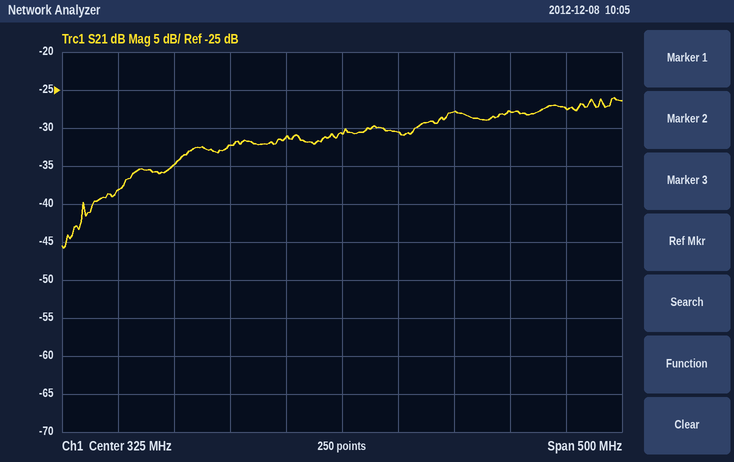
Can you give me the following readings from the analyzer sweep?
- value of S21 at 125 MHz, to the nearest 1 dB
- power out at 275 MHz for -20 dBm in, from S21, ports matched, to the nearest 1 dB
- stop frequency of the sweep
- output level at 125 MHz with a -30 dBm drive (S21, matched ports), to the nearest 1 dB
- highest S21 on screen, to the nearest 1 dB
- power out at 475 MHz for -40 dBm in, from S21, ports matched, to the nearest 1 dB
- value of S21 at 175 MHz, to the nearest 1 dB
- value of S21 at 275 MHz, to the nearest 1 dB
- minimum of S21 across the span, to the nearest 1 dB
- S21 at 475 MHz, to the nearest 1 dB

-38 dB
-51 dBm
575 MHz
-68 dBm
-26 dB
-68 dBm
-35 dB
-31 dB
-46 dB
-28 dB
